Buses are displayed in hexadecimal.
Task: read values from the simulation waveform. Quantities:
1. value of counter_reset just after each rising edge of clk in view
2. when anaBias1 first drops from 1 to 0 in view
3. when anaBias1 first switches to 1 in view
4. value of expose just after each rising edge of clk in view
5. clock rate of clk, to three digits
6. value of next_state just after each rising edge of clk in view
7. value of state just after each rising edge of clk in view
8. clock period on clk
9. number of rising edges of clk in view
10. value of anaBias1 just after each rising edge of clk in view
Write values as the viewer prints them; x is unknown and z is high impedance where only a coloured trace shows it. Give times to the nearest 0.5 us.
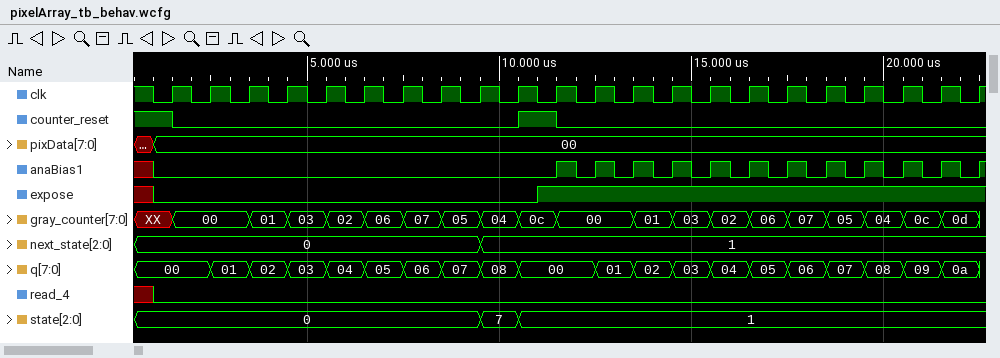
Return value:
0 0 0 0 0 0 0 0 0 1 0 0 0 0 0 0 0 0 0 0 0 0
12 us
11.5 us
0 0 0 0 0 0 0 0 0 0 1 1 1 1 1 1 1 1 1 1 1 1
1.00 MHz
0, 0, 0, 0, 0, 0, 0, 0, 1, 1, 1, 1, 1, 1, 1, 1, 1, 1, 1, 1, 1, 1
0, 0, 0, 0, 0, 0, 0, 0, 7, 1, 1, 1, 1, 1, 1, 1, 1, 1, 1, 1, 1, 1
1 us
22
0 0 0 0 0 0 0 0 0 0 1 1 1 1 1 1 1 1 1 1 1 1
